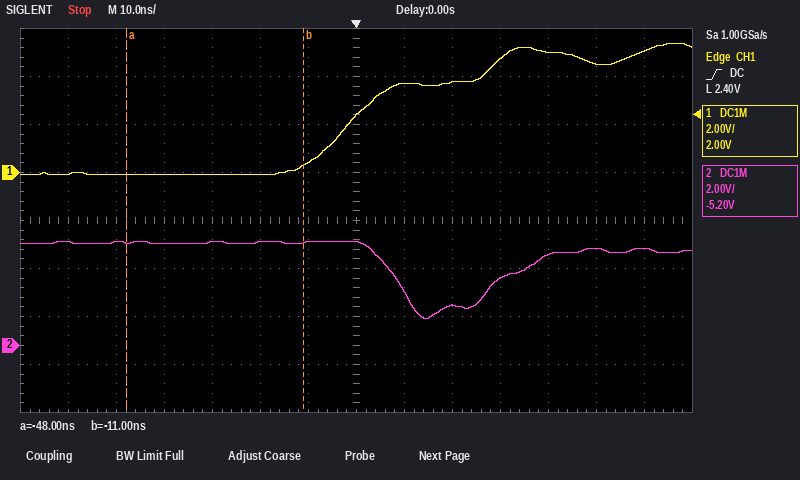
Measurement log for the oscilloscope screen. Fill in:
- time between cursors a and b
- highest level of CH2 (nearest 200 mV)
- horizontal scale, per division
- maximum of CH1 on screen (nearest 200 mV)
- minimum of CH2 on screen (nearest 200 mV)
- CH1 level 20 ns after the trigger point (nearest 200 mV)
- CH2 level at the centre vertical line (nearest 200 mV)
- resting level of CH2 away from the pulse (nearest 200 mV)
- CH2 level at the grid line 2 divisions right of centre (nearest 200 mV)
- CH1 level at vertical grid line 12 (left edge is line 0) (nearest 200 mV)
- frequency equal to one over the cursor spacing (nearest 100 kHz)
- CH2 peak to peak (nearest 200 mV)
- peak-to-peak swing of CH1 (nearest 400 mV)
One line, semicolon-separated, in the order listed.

37 ns; 4.4 V; 10 ns; 5.4 V; 1.2 V; 3.8 V; 4.4 V; 4.2 V; 1.6 V; 4.6 V; 27.0 MHz; 3.2 V; 5.6 V
